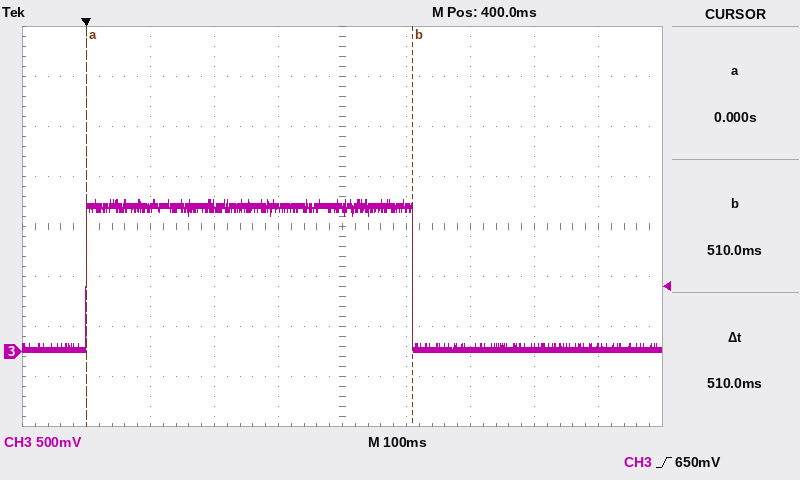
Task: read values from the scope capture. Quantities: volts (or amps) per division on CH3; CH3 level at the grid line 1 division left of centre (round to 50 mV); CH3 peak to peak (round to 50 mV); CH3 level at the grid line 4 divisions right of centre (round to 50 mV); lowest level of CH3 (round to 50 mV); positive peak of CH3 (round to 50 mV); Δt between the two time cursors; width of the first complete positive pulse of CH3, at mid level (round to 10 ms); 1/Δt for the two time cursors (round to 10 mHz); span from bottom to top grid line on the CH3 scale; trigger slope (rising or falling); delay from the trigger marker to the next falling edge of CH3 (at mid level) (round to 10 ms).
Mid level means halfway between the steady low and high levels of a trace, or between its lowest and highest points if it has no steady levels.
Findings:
500 mV
1.45 V
1.50 V
50 mV
0 mV
1.50 V
510 ms
510 ms
1.96 Hz
4 V
rising
510 ms
